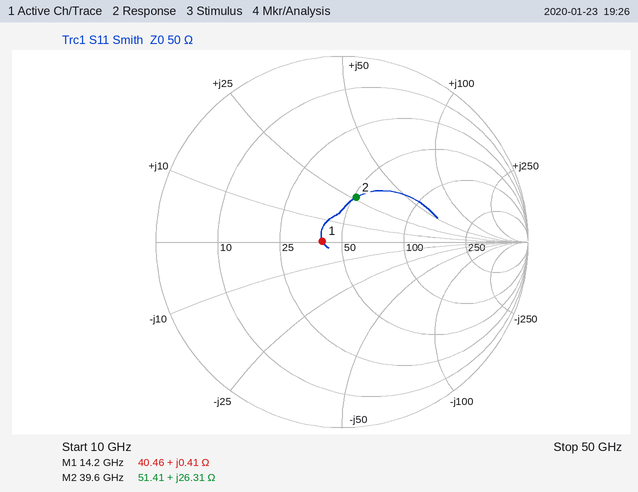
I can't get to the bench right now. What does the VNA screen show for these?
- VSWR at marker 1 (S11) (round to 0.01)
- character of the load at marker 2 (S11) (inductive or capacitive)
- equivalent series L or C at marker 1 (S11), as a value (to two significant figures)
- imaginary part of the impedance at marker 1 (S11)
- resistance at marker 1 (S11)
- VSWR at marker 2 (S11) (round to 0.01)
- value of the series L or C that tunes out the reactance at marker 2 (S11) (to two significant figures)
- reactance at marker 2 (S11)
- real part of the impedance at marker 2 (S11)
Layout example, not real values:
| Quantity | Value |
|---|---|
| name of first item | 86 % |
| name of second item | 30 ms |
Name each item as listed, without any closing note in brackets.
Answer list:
| Quantity | Value |
|---|---|
| VSWR at marker 1 (S11) | 1.24 |
| character of the load at marker 2 (S11) | inductive |
| equivalent series L or C at marker 1 (S11), as a value | 4.6 pH |
| imaginary part of the impedance at marker 1 | +0.41 Ω |
| resistance at marker 1 | 40.46 Ω |
| VSWR at marker 2 (S11) | 1.67 |
| value of the series L or C that tunes out the reactance at marker 2 (S11) | 150 fF |
| reactance at marker 2 | +26.31 Ω |
| real part of the impedance at marker 2 | 51.41 Ω |
